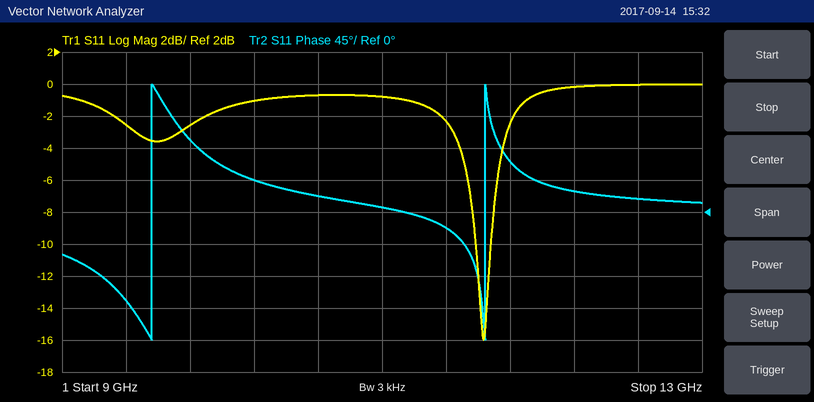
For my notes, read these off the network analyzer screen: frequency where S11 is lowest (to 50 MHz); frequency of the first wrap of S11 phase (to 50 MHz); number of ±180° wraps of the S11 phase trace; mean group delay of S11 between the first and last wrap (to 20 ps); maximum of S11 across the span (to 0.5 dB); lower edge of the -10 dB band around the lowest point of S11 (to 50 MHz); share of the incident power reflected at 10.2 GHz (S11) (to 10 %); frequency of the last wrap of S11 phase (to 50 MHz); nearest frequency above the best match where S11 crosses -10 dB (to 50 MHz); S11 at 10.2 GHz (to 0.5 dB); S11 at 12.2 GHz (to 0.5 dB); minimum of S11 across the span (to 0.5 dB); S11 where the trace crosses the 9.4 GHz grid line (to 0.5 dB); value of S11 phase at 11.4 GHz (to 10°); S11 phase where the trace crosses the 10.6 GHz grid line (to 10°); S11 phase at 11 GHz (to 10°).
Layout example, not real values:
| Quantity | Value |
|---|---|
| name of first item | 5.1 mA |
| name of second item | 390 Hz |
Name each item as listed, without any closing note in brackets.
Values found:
| Quantity | Value |
|---|---|
| frequency where S11 is lowest | 11.65 GHz |
| frequency of the first wrap of S11 phase | 9.55 GHz |
| number of ±180° wraps of the S11 phase trace | 2 |
| mean group delay of S11 between the first and last wrap | 480 ps |
| maximum of S11 across the span | 0.0 dB |
| lower edge of the -10 dB band around the lowest point of S11 | 11.60 GHz |
| share of the incident power reflected at 10.2 GHz (S11) | 80 % |
| frequency of the last wrap of S11 phase | 11.65 GHz |
| nearest frequency above the best match where S11 crosses -10 dB | 11.70 GHz |
| S11 at 10.2 GHz | -1.0 dB |
| S11 at 12.2 GHz | 0.0 dB |
| minimum of S11 across the span | -16.0 dB |
| S11 where the trace crosses the 9.4 GHz grid line | -2.5 dB |
| value of S11 phase at 11.4 GHz | -20° |
| S11 phase where the trace crosses the 10.6 GHz grid line | 20° |
| S11 phase at 11 GHz | 10° |
